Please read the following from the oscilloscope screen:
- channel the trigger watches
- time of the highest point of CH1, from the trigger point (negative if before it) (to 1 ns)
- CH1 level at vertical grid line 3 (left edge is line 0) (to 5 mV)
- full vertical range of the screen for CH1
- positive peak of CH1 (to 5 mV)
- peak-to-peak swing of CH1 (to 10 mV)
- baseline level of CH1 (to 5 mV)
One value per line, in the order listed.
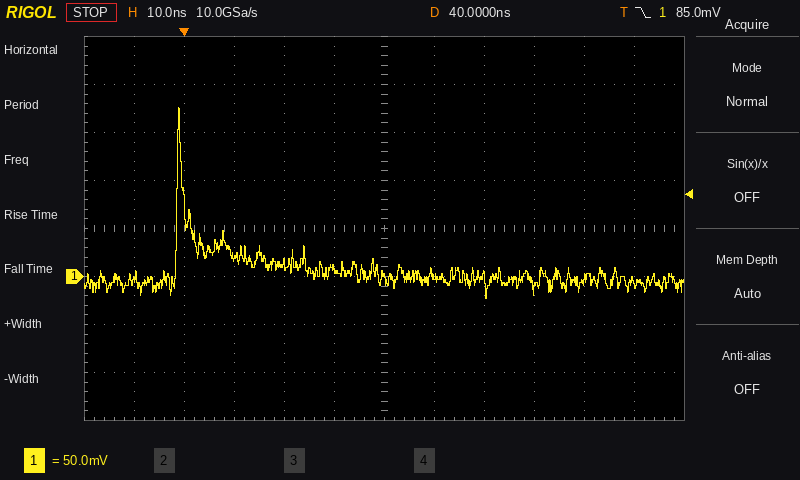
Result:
CH1
-1 ns
20 mV
400 mV
175 mV
200 mV
0 mV
